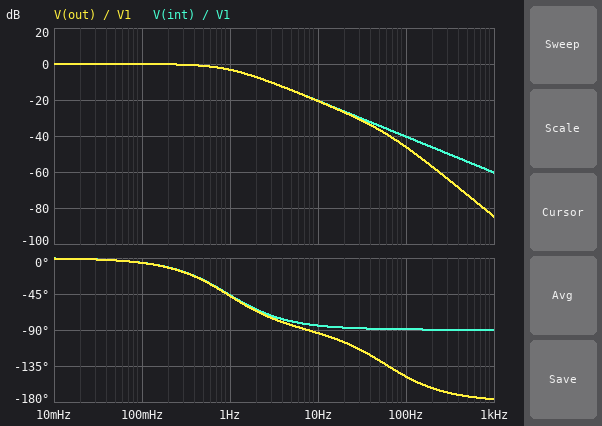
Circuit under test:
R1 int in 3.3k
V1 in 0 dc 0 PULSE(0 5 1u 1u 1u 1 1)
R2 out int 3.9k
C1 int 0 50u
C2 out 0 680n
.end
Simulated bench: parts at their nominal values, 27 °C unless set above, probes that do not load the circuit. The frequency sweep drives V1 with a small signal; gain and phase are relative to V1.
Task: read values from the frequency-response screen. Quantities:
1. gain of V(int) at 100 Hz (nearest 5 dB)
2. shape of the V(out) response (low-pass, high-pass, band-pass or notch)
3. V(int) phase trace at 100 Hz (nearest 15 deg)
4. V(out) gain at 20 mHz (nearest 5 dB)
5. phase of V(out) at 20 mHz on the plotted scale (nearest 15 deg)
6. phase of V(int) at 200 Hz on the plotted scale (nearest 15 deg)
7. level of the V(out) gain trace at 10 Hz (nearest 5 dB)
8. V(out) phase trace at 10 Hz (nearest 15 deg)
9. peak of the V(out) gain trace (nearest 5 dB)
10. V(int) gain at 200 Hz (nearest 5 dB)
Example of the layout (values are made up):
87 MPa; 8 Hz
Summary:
-40 dB; low-pass; -90 deg; 0 dB; 0 deg; -90 deg; -20 dB; -90 deg; 0 dB; -45 dB
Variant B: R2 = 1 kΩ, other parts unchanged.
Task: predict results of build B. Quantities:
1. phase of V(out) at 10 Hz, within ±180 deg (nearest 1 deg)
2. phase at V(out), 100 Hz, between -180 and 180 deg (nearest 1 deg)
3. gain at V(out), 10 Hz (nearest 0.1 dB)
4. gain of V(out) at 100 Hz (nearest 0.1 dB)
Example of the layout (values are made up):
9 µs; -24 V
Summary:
-87 deg; -112 deg; -20.5 dB; -41.1 dB
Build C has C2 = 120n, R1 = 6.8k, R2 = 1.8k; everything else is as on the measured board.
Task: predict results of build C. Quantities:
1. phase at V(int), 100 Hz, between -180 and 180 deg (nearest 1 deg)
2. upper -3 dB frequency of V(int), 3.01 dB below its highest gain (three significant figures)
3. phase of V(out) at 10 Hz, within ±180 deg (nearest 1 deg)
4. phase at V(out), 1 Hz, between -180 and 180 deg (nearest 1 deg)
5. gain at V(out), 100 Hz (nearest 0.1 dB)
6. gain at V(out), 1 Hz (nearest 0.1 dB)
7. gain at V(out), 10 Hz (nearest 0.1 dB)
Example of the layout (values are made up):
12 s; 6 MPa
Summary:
-90 deg; 467 mHz; -88 deg; -65 deg; -46.7 dB; -7.5 dB; -26.6 dB
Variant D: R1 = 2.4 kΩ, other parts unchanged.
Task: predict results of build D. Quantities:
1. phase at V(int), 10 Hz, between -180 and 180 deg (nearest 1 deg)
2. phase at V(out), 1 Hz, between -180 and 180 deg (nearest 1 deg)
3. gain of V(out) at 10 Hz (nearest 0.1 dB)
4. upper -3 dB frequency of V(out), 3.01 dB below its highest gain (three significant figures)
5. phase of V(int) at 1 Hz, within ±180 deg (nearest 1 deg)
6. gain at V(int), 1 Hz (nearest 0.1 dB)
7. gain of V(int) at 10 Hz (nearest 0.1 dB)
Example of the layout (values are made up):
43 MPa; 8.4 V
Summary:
-82 deg; -38 deg; -17.9 dB; 1.31 Hz; -37 deg; -2.0 dB; -17.7 dB
